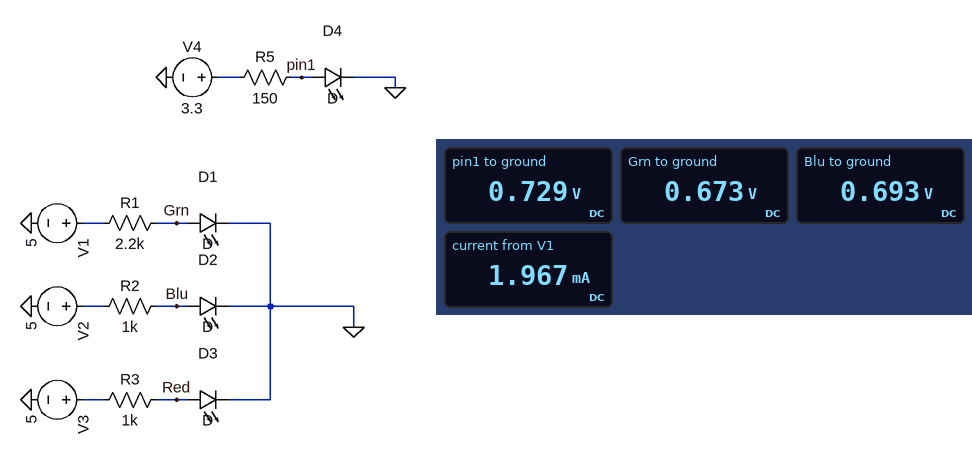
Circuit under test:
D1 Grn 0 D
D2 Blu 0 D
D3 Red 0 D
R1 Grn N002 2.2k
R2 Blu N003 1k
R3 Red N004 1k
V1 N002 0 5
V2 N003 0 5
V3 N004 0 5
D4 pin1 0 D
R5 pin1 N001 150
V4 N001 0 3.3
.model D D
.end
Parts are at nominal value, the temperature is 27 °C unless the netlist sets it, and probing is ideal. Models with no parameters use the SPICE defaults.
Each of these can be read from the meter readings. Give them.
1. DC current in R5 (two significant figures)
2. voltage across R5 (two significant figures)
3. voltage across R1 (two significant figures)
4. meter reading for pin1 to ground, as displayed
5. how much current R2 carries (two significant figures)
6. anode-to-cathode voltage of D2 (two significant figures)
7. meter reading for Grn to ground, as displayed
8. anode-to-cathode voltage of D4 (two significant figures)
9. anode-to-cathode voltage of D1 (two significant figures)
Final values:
17 mA
2.6 V
4.3 V
0.729 V
4.3 mA
690 mV
0.673 V
730 mV
670 mV
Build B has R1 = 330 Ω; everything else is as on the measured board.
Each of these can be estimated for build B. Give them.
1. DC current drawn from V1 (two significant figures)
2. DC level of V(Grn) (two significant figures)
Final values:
13 mA
720 mV
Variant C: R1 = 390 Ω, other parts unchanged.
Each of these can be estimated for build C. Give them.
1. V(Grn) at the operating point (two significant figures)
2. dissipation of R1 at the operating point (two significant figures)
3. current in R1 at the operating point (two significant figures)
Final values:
720 mV
47 mW
11 mA
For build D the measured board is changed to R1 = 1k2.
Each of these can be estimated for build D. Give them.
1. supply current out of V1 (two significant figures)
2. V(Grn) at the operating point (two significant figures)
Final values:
3.6 mA
690 mV
